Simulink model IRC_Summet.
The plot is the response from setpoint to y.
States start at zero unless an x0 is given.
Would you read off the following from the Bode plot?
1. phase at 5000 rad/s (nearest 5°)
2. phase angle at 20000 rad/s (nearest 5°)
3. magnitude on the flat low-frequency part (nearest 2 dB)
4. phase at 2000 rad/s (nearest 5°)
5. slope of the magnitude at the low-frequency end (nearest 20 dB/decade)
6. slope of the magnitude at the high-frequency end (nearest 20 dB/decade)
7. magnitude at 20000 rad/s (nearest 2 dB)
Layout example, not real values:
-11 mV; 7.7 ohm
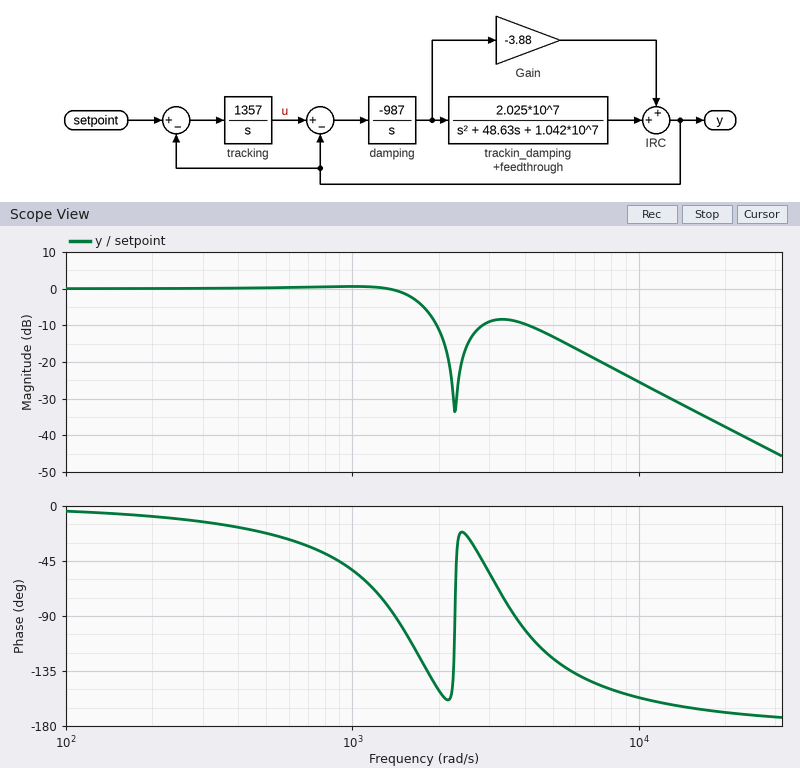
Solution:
-125°; -170°; 0 dB; -150°; 0 dB/decade; -40 dB/decade; -38 dB
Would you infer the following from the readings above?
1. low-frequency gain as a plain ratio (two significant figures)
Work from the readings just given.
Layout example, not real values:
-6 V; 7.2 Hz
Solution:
1.0
